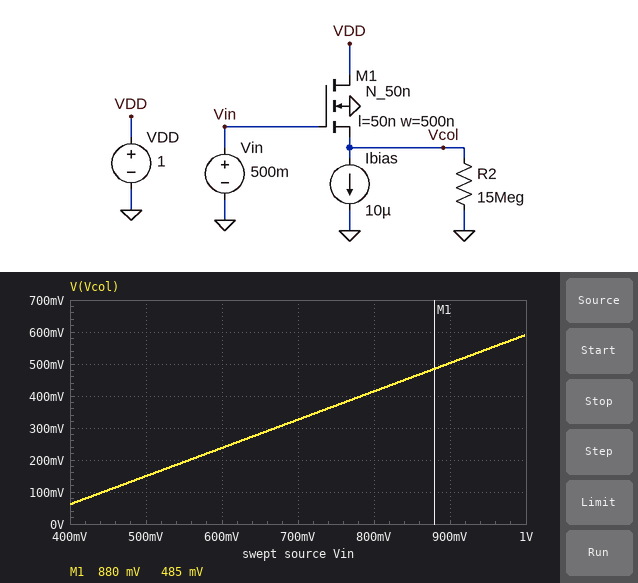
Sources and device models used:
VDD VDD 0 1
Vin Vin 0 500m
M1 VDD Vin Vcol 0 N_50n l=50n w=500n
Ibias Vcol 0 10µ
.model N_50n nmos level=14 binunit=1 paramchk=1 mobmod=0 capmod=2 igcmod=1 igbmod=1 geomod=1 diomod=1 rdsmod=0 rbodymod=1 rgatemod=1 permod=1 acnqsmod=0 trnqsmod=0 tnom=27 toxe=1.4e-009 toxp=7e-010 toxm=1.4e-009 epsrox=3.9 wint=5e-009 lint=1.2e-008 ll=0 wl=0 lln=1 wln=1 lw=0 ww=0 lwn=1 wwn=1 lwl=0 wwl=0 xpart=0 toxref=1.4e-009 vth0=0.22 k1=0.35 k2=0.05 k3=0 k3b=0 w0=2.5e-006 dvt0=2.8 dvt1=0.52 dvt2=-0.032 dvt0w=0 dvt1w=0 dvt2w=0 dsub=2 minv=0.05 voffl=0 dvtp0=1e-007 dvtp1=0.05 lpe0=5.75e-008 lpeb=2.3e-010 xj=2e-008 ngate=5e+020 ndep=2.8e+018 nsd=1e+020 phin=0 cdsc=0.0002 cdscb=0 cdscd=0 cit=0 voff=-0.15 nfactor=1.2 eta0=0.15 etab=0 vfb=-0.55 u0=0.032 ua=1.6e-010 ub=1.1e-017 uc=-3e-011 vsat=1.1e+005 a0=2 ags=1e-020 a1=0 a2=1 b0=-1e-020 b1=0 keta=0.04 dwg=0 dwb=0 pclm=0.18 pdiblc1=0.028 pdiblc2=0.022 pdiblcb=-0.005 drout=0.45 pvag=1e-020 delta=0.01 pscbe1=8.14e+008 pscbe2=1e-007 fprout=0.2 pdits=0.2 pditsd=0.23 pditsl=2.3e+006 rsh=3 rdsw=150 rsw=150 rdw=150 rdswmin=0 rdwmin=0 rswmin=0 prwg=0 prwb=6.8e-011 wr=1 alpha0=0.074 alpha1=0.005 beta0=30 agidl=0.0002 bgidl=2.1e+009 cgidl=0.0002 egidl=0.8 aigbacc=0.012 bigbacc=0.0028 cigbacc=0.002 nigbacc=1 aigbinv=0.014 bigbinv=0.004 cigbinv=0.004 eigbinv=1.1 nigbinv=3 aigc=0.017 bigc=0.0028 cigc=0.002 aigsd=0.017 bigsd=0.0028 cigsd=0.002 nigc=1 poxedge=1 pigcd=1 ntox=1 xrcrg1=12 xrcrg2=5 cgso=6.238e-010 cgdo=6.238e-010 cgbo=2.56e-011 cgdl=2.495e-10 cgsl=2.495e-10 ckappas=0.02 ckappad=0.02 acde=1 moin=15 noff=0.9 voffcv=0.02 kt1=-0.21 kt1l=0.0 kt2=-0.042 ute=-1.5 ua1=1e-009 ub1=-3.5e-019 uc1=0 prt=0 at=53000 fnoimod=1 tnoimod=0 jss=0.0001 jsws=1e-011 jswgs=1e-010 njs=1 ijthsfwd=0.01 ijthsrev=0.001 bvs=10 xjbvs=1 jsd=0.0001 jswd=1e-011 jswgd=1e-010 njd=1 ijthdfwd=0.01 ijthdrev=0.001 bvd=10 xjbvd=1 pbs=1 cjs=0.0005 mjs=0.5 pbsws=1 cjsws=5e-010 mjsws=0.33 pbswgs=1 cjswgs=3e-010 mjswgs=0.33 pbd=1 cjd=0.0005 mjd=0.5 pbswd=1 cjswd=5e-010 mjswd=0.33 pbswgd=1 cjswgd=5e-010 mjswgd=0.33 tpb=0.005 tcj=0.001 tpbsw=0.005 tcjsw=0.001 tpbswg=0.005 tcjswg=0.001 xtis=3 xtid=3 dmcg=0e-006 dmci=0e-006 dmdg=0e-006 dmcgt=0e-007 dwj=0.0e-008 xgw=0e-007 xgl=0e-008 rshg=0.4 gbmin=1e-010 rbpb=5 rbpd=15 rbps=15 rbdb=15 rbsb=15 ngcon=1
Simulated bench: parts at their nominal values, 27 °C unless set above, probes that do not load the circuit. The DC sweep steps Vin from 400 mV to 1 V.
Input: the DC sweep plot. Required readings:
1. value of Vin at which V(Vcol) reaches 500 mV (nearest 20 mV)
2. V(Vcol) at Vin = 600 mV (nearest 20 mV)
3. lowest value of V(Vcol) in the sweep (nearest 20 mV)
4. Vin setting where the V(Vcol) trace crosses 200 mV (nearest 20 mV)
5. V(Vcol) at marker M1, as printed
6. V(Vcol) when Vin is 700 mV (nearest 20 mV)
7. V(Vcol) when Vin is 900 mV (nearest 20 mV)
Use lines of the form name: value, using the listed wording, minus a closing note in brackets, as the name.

value of Vin at which V(Vcol) reaches 500 mV: 900 mV
V(Vcol) at Vin = 600 mV: 240 mV
lowest value of V(Vcol) in the sweep: 60 mV
Vin setting where the V(Vcol) trace crosses 200 mV: 560 mV
V(Vcol) at marker M1, as printed: 485 mV
V(Vcol) when Vin is 700 mV: 320 mV
V(Vcol) when Vin is 900 mV: 500 mV
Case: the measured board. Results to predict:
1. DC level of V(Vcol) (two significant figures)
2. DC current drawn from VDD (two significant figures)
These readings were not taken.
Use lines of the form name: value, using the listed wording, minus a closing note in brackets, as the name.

DC level of V(Vcol): 150 mV
DC current drawn from VDD: 10 µA
